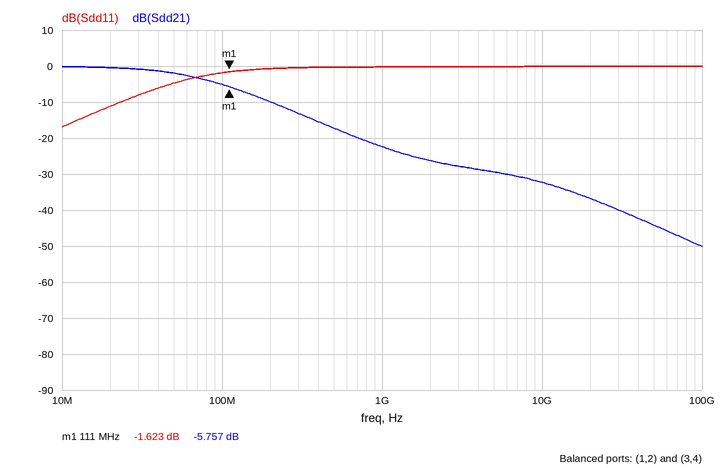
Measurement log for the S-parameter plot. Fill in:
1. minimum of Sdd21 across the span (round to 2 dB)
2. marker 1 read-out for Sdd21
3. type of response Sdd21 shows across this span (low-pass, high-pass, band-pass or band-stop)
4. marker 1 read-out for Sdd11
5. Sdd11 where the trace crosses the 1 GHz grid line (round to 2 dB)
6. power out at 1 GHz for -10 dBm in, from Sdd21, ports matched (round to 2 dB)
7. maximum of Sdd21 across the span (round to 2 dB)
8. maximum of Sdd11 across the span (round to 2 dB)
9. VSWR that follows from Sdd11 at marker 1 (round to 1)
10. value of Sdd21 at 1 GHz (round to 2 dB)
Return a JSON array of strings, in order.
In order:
["-50 dB", "-5.757 dB", "low-pass", "-1.623 dB", "0 dB", "-32 dBm", "0 dB", "0 dB", "11", "-22 dB"]
